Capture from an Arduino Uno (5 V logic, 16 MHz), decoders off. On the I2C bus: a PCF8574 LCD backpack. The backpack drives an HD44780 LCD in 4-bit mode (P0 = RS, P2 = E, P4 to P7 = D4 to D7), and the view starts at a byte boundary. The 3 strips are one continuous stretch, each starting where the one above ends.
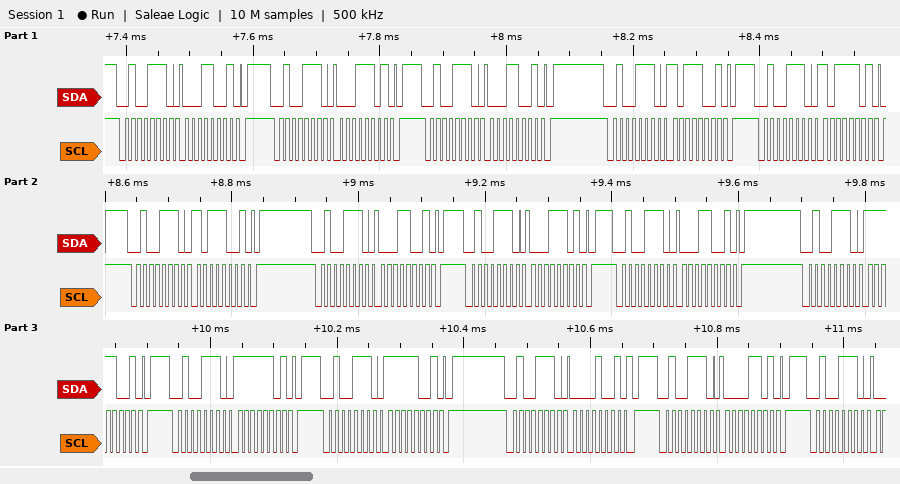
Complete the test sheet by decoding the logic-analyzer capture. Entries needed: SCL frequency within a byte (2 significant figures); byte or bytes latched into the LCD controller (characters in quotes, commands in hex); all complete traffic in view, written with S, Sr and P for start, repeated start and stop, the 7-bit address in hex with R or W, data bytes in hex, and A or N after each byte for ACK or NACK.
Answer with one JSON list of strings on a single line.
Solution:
["100 kHz", "data 0x1B data 0x1F", "S 27W A 19 A P S 27W A 1D A P S 27W A 19 A P S 27W A B9 A P S 27W A BD A P S 27W A B9 A P S 27W A 19 A P S 27W A 1D A P S 27W A 19 A P S 27W A F9 A P S 27W A FD A P S 27W A F9 A P S 27W A 09 A P S 27W A 0D A P S 27W A"]
